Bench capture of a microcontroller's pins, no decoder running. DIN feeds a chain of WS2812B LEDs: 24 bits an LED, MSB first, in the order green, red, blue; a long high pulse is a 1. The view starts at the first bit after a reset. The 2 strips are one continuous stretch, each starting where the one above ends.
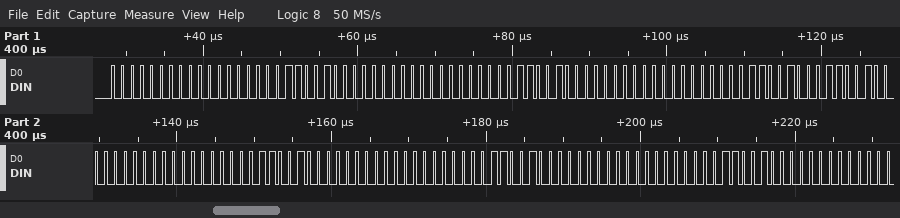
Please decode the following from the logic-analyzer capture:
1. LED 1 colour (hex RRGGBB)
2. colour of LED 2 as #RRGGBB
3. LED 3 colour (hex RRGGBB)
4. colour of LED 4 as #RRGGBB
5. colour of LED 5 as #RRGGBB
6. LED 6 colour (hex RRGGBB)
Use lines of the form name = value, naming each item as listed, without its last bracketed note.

LED 1 colour = #000032
colour of LED 2 as #RRGGBB = #000032
LED 3 colour = #000032
colour of LED 4 as #RRGGBB = #003200
colour of LED 5 as #RRGGBB = #003200
LED 6 colour = #003200
